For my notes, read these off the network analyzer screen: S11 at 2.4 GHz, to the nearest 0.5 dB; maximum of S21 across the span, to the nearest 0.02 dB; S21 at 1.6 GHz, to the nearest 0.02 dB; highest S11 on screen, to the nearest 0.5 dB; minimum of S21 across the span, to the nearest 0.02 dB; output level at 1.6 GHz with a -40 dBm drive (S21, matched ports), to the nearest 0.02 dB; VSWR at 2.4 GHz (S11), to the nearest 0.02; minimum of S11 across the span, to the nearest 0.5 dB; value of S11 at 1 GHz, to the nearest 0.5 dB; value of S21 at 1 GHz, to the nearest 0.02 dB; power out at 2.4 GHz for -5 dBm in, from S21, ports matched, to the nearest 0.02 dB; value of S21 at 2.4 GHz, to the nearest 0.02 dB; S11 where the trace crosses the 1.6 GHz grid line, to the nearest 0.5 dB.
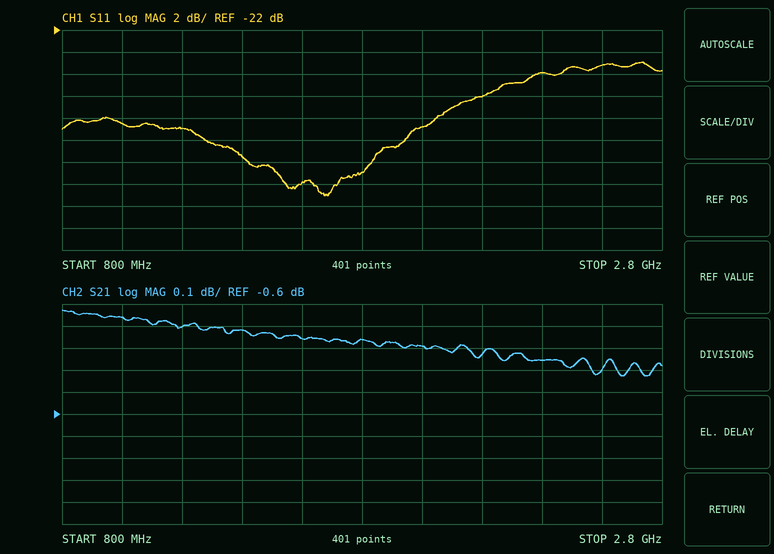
-26.0 dB
-0.12 dB
-0.26 dB
-25.0 dB
-0.42 dB
-40.26 dBm
1.10
-37.0 dB
-30.5 dB
-0.16 dB
-5.36 dBm
-0.36 dB
-36.0 dB
